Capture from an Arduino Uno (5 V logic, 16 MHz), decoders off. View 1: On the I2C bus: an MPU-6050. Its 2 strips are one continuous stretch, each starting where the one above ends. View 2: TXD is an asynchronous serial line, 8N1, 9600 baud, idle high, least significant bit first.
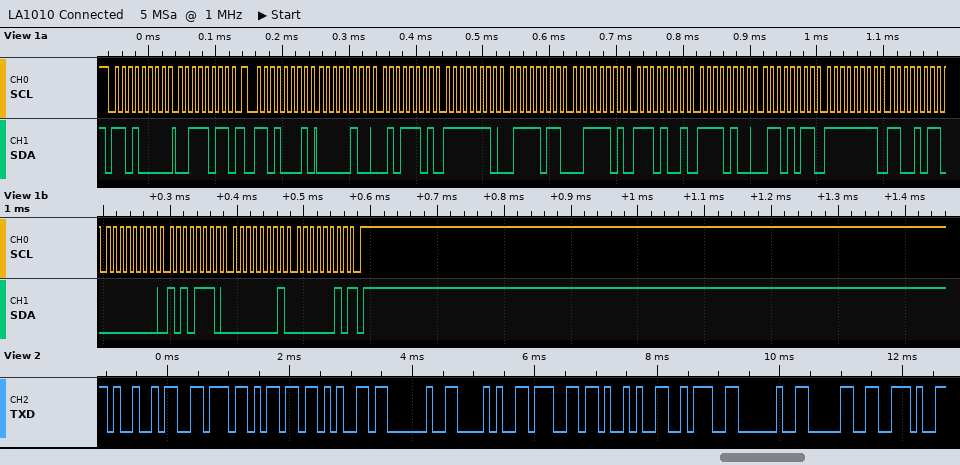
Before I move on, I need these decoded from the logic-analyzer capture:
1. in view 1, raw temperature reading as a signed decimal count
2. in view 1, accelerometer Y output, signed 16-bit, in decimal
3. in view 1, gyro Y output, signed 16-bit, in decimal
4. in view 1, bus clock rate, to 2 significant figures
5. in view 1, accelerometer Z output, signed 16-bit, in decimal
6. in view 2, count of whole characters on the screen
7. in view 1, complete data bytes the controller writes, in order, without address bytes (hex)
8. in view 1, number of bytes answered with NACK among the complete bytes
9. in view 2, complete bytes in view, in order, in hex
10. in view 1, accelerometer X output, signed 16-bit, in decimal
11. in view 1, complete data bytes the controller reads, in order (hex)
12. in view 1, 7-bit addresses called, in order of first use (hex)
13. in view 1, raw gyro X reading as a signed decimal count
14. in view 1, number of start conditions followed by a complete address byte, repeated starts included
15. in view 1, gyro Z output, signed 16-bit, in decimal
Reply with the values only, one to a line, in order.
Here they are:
-2965
-389
174
100 kHz
15849
12
3B
1
49 76 6D 65 20 28 67 29 3A 20 30 2E
1117
04 5D FE 7B 3D E9 F4 6B FF CB 00 AE 01 02
0x68
-53
2
258
